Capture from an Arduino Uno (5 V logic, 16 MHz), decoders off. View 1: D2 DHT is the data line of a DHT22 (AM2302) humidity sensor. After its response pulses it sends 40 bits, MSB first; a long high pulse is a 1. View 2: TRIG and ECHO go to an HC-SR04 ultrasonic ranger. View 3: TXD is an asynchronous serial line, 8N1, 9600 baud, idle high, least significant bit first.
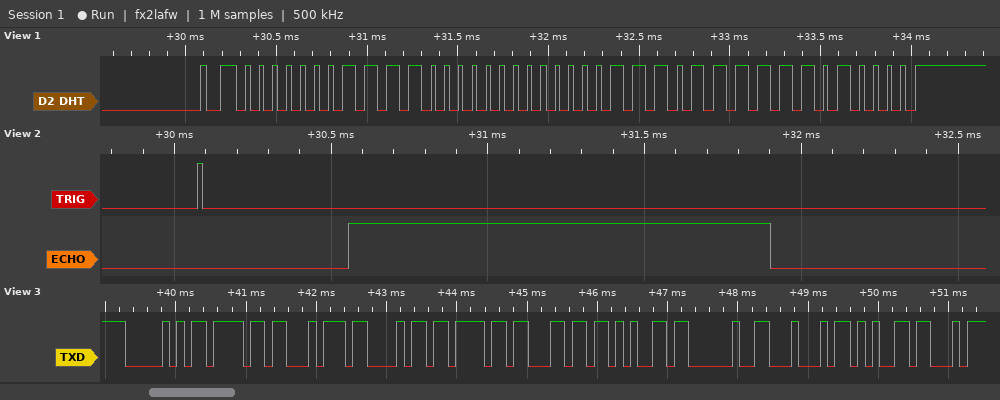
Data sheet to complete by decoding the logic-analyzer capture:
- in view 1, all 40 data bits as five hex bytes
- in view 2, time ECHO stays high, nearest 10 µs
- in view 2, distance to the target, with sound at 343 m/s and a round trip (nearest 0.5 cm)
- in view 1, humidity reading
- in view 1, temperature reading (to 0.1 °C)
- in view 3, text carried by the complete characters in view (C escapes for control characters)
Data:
01 E0 00 EF D0
1350 µs
23 cm
48.0 %
23.9 °C
"Pothole De"
